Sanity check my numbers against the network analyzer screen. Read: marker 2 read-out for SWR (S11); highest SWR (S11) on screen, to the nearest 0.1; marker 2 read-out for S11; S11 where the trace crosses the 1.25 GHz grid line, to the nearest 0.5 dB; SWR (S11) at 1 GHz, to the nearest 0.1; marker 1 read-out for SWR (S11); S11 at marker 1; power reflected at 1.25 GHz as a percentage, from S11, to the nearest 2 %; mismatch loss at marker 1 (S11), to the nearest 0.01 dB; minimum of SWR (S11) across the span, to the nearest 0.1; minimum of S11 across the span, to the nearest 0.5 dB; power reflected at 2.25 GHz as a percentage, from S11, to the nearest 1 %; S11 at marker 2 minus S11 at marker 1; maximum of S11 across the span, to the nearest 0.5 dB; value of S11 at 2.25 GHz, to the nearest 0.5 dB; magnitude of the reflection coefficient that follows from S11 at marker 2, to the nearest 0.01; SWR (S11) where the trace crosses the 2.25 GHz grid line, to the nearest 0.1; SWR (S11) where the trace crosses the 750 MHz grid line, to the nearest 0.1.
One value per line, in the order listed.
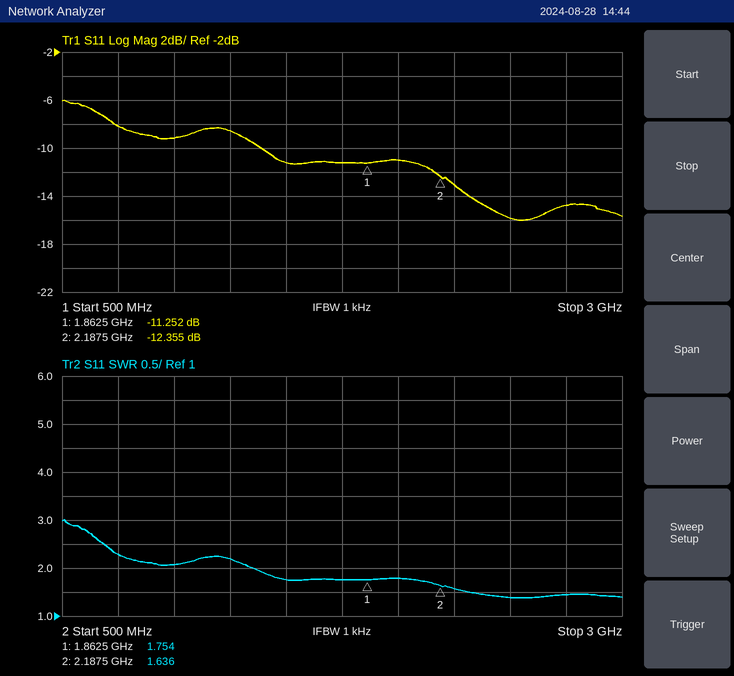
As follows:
1.636
3.0
-12.355 dB
-8.5 dB
2.1
1.754
-11.252 dB
14 %
0.34 dB
1.4
-16.0 dB
5 %
-1.103 dB
-6.0 dB
-13.0 dB
0.24
1.6
2.3
